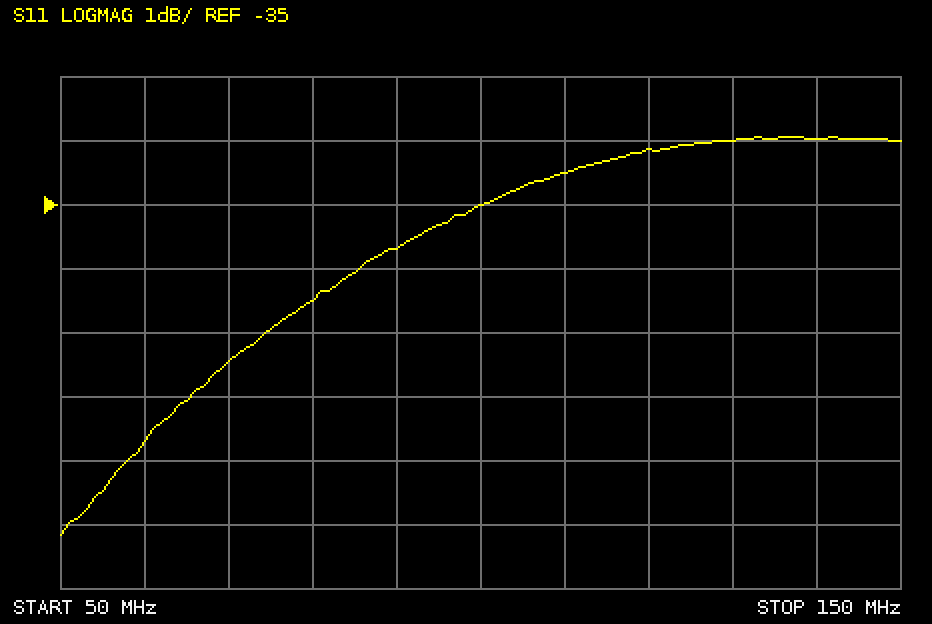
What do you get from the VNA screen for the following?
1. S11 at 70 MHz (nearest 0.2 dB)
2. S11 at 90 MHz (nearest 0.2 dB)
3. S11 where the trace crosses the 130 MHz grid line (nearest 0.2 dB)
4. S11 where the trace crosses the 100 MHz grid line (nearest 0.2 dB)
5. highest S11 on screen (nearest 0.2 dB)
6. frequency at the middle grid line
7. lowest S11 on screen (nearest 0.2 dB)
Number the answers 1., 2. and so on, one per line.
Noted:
1. -37.4 dB
2. -35.6 dB
3. -34.0 dB
4. -35.0 dB
5. -34.0 dB
6. 100 MHz
7. -40.2 dB
